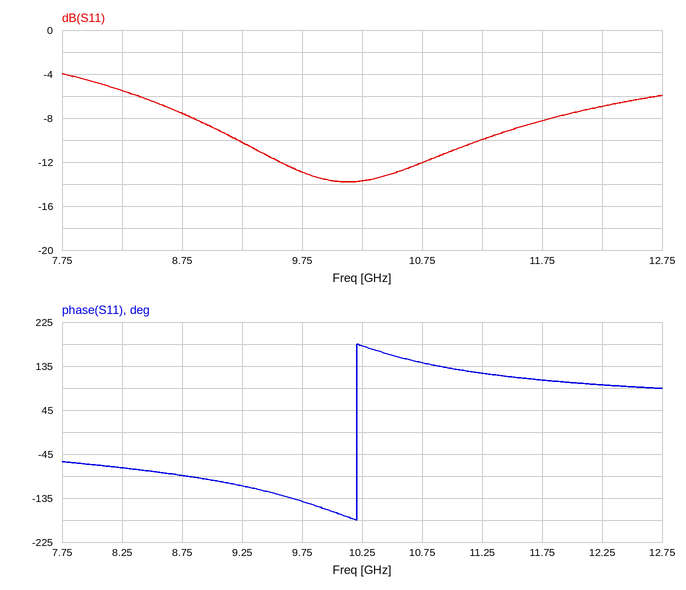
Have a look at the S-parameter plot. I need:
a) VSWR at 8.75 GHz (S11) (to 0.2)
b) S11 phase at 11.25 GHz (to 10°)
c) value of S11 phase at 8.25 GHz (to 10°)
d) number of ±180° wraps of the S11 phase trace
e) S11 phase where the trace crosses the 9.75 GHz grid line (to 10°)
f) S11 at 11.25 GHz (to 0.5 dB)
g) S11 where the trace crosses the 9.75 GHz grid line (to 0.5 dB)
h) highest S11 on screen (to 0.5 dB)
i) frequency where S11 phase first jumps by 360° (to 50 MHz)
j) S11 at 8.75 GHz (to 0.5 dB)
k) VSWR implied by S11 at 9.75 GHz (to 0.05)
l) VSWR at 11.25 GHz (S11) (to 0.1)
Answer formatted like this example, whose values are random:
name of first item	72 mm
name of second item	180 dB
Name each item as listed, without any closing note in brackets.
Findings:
VSWR at 8.75 GHz (S11)	2.4
S11 phase at 11.25 GHz	120°
value of S11 phase at 8.25 GHz	-70°
number of ±180° wraps of the S11 phase trace	1
S11 phase where the trace crosses the 9.75 GHz grid line	-140°
S11 at 11.25 GHz	-10.0 dB
S11 where the trace crosses the 9.75 GHz grid line	-13.0 dB
highest S11 on screen	-4.0 dB
frequency where S11 phase first jumps by 360°	10.20 GHz
S11 at 8.75 GHz	-7.5 dB
VSWR implied by S11 at 9.75 GHz	1.60
VSWR at 11.25 GHz (S11)	1.9
